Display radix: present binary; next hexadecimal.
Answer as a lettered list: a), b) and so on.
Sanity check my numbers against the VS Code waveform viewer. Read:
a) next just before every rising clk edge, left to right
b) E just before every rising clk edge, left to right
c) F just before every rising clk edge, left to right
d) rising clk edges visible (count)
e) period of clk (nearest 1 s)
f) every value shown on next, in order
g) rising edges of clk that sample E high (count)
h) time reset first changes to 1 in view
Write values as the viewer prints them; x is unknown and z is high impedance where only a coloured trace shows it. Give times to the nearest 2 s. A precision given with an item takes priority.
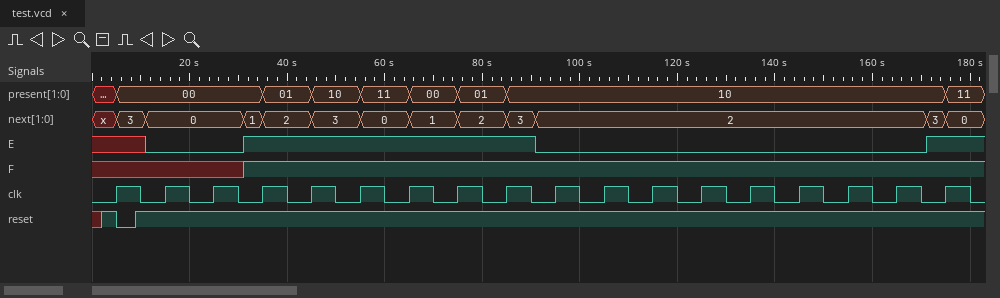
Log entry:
a) x, 0, 0, 1, 2, 3, 0, 1, 2, 2, 2, 2, 2, 2, 2, 2, 2, 3
b) x 0 0 1 1 1 1 1 1 0 0 0 0 0 0 0 0 1
c) x x x 1 1 1 1 1 1 1 1 1 1 1 1 1 1 1
d) 18
e) 10 s
f) x, 3, 0, 1, 2, 3, 0, 1, 2, 3, 2, 3, 0
g) 7
h) 2 s
